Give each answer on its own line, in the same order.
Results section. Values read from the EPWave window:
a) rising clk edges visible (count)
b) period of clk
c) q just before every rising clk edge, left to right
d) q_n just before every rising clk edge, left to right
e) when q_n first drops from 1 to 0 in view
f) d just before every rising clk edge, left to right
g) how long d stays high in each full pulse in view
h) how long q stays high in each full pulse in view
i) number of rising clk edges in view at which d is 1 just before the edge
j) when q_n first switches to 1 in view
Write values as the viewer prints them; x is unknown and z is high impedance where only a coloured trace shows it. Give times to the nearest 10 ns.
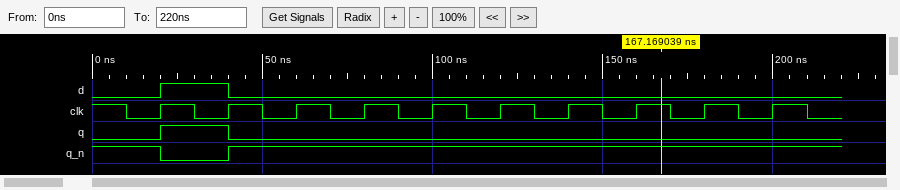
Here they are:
10
20 ns
0 1 0 0 0 0 0 0 0 0
1 0 1 1 1 1 1 1 1 1
20 ns
0 1 0 0 0 0 0 0 0 0
20 ns
20 ns
1
40 ns
